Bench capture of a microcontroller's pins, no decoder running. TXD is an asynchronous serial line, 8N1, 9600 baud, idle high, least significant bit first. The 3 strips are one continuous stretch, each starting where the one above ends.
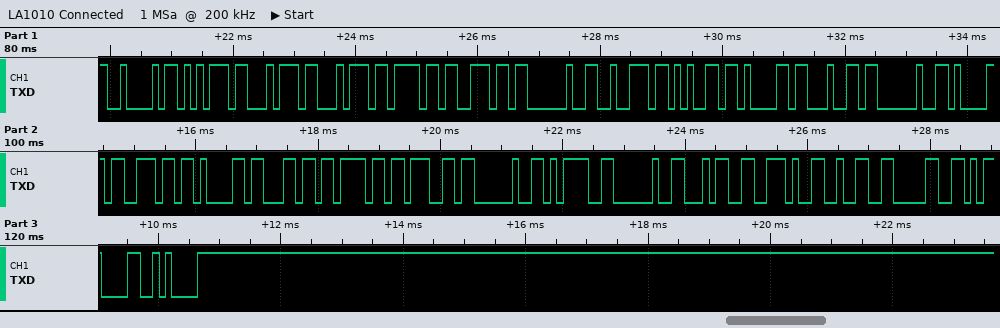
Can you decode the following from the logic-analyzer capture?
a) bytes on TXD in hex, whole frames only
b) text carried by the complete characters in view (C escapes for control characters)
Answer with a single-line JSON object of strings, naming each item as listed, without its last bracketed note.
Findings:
{"bytes on TXD in hex, whole frames only": "42 75 74 74 6F 6E 20 72 65 61 64 20 61 6E 61 6C 6F 67 20 3D 20 34 2E 32 30 0D 0A", "text carried by the complete characters in view": "\"Button read analog = 4.20\\r\\n\""}
